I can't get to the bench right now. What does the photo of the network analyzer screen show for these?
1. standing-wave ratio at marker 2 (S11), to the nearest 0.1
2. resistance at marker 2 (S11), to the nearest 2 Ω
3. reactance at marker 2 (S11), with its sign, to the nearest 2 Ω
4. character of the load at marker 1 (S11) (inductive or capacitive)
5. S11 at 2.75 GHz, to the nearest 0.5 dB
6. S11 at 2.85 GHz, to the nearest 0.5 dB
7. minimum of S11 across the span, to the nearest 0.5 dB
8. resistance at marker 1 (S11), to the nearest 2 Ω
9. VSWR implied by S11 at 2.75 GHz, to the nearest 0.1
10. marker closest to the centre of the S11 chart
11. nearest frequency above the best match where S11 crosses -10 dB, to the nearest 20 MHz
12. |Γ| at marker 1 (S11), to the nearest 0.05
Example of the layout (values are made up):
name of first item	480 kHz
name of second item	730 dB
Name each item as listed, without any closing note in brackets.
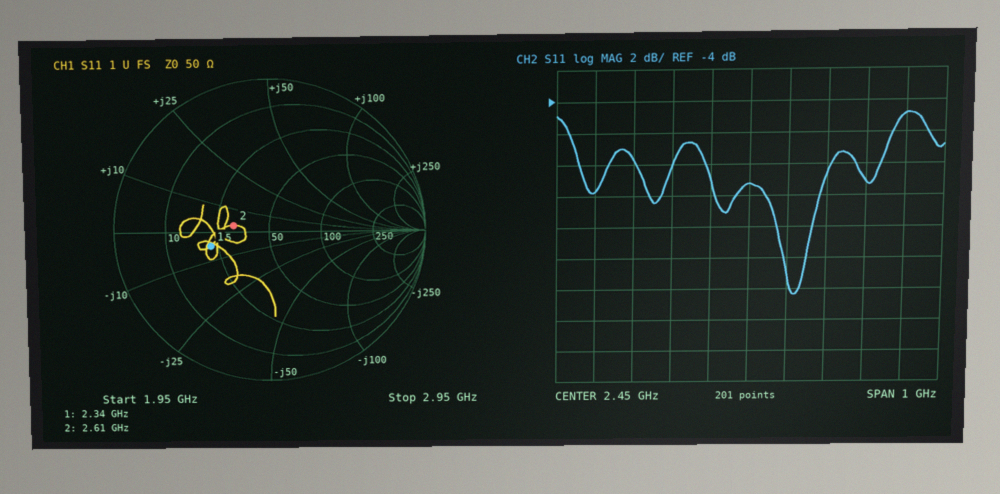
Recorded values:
standing-wave ratio at marker 2 (S11), to the nearest 0.1	1.6
resistance at marker 2 (S11), to the nearest 2 Ω	32 Ω
reactance at marker 2 (S11), with its sign, to the nearest 2 Ω	+2 Ω
character of the load at marker 1 (S11)	capacitive
S11 at 2.75 GHz, to the nearest 0.5 dB	-9.0 dB
S11 at 2.85 GHz, to the nearest 0.5 dB	-5.0 dB
minimum of S11 across the span, to the nearest 0.5 dB	-16.5 dB
resistance at marker 1 (S11), to the nearest 2 Ω	22 Ω
VSWR implied by S11 at 2.75 GHz, to the nearest 0.1	2.1
marker closest to the centre of the S11 chart	marker 2
nearest frequency above the best match where S11 crosses -10 dB, to the nearest 20 MHz	2.64 GHz
|Γ| at marker 1 (S11), to the nearest 0.05	0.40
